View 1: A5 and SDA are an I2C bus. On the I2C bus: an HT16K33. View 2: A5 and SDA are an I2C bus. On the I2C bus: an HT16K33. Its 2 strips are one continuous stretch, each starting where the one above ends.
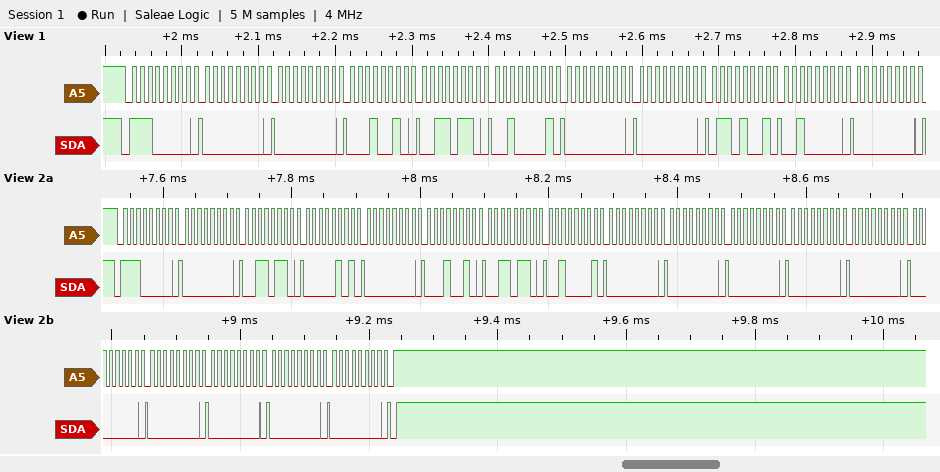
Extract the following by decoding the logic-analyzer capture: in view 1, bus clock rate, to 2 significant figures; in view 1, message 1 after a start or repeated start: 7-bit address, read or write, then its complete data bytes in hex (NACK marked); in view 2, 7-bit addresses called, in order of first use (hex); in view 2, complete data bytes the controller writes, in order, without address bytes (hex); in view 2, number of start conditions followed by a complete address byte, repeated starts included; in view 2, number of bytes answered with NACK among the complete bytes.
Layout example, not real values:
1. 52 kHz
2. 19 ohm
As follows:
1. 100 kHz
2. 0x70 write: 00 00 12 36 21 00 00 69 20 00
3. 0x70
4. 00 36 05 00 12 36 21 00 00 00 00 00 00 00 00 00 00
5. 1
6. 0
